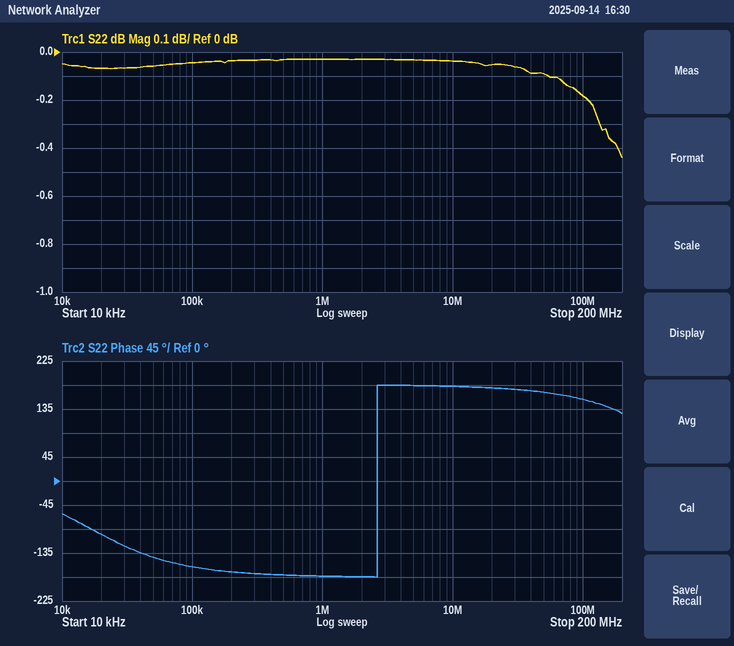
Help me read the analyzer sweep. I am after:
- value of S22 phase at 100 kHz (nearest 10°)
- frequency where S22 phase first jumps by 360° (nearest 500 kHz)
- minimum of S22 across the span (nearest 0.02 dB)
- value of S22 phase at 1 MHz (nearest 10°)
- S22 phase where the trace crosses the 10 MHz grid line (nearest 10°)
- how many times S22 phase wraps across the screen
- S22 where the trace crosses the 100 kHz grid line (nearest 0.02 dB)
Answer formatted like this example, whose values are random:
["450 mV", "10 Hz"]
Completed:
["-160°", "2.5 MHz", "-0.44 dB", "-180°", "180°", "1", "-0.04 dB"]
